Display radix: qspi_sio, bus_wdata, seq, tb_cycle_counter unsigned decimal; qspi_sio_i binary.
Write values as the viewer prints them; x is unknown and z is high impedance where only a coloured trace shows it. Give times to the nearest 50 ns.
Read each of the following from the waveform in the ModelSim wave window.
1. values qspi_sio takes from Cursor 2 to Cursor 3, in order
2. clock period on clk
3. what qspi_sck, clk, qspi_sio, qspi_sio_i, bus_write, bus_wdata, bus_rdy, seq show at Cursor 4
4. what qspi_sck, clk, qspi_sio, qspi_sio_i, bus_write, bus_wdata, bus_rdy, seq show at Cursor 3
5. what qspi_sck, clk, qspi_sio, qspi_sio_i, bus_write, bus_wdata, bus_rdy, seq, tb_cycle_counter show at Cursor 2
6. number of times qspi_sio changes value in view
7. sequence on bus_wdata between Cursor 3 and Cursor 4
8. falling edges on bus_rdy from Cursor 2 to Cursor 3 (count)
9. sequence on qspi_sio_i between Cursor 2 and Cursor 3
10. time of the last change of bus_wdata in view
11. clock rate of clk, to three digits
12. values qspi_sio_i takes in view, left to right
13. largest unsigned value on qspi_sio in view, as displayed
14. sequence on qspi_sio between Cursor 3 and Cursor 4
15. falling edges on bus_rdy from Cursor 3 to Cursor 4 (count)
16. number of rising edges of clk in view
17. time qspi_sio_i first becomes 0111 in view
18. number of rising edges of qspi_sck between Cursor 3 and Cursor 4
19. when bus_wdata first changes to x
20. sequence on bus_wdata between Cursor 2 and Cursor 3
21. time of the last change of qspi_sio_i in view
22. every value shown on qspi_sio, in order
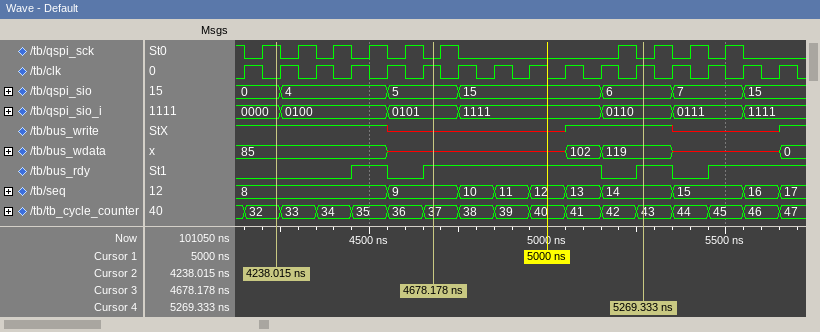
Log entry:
0, 4, 5
100 ns
qspi_sck=0, clk=1, qspi_sio=6, qspi_sio_i=0110, bus_write=1, bus_wdata=119, bus_rdy=1, seq=14
qspi_sck=0, clk=1, qspi_sio=5, qspi_sio_i=0101, bus_write=x, bus_wdata=x, bus_rdy=1, seq=9
qspi_sck=1, clk=0, qspi_sio=0, qspi_sio_i=0000, bus_write=1, bus_wdata=85, bus_rdy=0, seq=8, tb_cycle_counter=32
6
x, 102, 119
1
0000, 0100, 0101
5650 ns
10.0 MHz
0000, 0100, 0101, 1111, 0110, 0111, 1111
15
5, 15, 6
1
16
5350 ns
2
4550 ns
85, x
5550 ns
0, 4, 5, 15, 6, 7, 15
